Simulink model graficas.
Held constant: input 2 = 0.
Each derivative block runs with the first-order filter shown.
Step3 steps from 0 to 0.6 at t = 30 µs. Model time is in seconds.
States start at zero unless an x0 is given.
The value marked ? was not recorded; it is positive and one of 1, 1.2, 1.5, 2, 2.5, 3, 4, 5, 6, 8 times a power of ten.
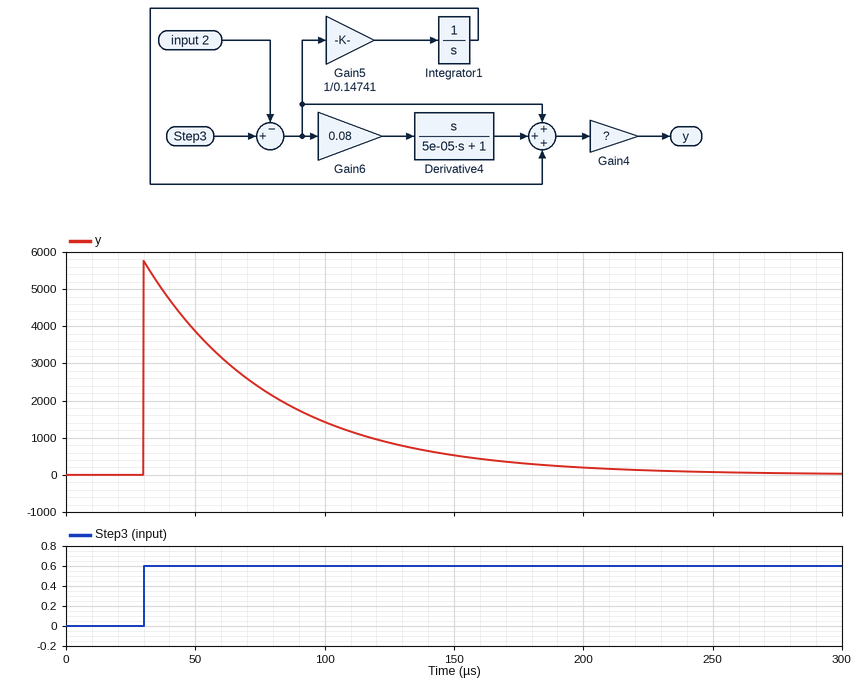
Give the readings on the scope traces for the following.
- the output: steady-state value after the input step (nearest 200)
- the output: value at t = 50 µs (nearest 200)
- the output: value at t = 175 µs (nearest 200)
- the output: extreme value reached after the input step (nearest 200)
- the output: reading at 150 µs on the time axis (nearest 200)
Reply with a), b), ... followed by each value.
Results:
a) 0
b) 3800
c) 400
d) 5800
e) 600
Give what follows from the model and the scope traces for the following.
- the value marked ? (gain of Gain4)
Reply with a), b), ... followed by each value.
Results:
a) 6
